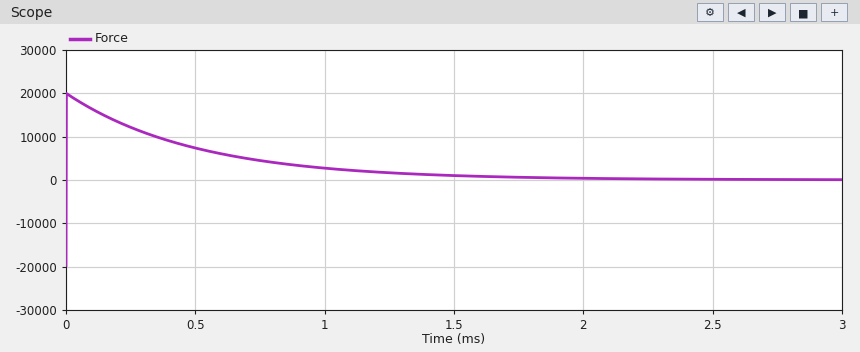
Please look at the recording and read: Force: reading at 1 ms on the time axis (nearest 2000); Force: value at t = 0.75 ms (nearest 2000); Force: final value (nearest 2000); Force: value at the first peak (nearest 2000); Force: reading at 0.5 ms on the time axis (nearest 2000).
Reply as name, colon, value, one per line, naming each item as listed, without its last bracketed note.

Force: reading at 1 ms on the time axis: 2000
Force: value at t = 0.75 ms: 4000
Force: final value: 0
Force: value at the first peak: 20000
Force: reading at 0.5 ms on the time axis: 8000
